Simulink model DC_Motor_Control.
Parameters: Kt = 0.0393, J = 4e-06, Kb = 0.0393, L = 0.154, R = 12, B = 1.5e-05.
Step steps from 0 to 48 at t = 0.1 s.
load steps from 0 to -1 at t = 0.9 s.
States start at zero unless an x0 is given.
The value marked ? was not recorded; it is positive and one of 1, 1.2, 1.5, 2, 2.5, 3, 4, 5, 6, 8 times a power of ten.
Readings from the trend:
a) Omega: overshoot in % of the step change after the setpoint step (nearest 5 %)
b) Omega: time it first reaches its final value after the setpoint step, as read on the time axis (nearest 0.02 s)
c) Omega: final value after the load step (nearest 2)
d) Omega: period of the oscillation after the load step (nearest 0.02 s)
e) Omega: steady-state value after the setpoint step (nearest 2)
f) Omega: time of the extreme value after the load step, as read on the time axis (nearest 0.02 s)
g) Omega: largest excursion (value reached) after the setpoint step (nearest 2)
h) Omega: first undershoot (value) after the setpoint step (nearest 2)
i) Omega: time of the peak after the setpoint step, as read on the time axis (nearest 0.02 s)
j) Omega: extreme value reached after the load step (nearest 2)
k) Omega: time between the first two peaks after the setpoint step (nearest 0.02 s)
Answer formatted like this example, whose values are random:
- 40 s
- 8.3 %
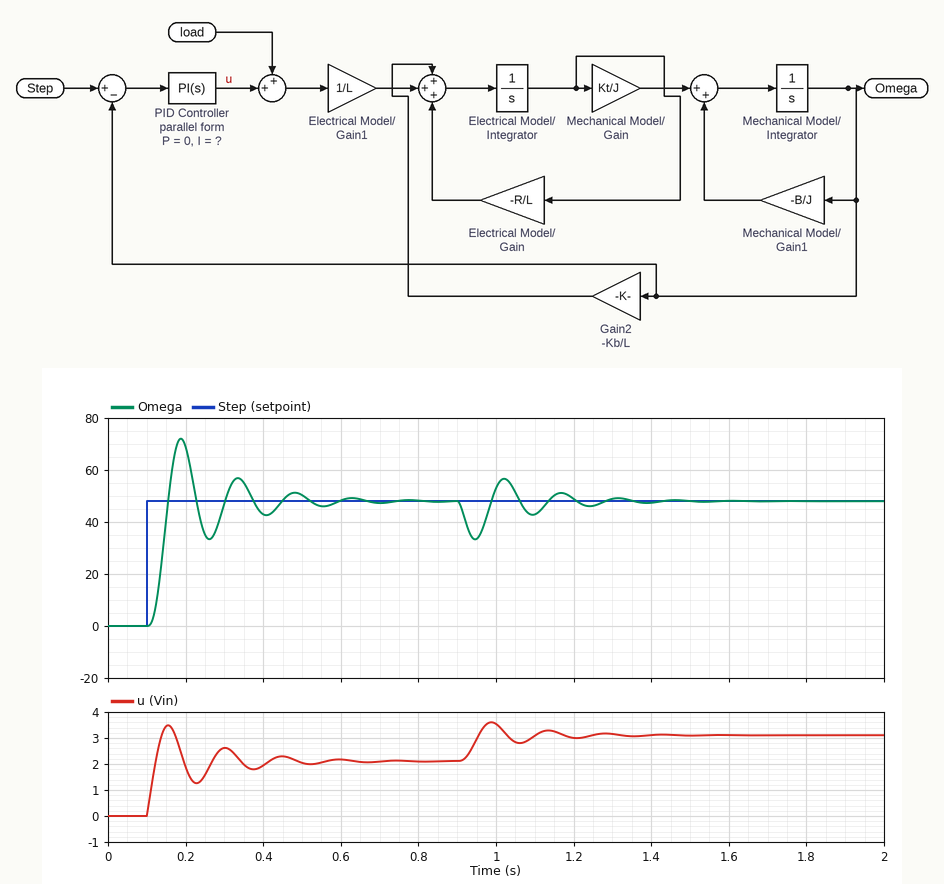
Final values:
- 50 %
- 0.16 s
- 48
- 0.14 s
- 48
- 0.94 s
- 72
- 34
- 0.18 s
- 34
- 0.14 s
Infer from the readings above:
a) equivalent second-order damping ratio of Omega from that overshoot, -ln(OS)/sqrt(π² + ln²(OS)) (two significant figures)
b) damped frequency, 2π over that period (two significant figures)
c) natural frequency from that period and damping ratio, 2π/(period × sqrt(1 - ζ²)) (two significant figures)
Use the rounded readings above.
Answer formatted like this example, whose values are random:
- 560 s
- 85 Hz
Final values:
- 0.22
- 45 rad/s
- 46 rad/s
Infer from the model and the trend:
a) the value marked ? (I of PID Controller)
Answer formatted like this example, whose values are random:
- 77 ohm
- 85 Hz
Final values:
- 2
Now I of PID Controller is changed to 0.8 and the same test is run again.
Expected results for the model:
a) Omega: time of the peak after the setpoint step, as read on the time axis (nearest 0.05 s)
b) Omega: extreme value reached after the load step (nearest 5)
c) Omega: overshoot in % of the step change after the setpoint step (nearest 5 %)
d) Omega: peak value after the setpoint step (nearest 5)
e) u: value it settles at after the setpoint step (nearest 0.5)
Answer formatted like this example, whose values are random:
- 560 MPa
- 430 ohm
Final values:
- 0.25 s
- 30
- 10 %
- 50
- 2.0
